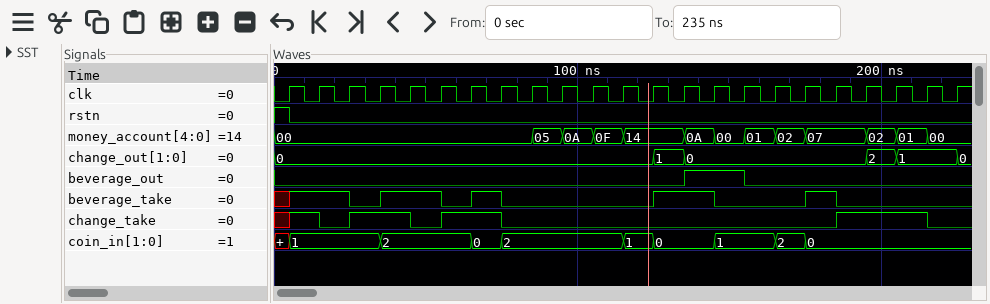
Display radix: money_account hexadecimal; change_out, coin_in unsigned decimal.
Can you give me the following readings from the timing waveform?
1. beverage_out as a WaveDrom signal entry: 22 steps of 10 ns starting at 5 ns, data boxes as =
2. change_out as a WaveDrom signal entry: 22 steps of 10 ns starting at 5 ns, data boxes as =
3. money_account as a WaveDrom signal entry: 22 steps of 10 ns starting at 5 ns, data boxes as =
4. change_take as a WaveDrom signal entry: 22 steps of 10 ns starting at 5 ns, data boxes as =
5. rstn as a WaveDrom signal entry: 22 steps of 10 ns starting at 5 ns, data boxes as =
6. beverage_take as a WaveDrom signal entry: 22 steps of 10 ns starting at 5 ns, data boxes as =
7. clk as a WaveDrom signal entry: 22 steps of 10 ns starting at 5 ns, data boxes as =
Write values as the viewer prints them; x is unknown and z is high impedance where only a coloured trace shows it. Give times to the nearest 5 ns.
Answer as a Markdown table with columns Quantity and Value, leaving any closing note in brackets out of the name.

| Quantity | Value |
|---|---|
| beverage_out as a WaveDrom signal entry: 22 steps of 10 ns starting at 5 ns, data boxes as = | {name: 'beverage_out', wave: '0............1.0......'} |
| change_out as a WaveDrom signal entry: 22 steps of 10 ns starting at 5 ns, data boxes as = | {name: 'change_out', wave: '=...........==.....==.', data: '0 1 0 2 1'} |
| money_account as a WaveDrom signal entry: 22 steps of 10 ns starting at 5 ns, data boxes as = | {name: 'money_account', wave: '=.......====.=====.===', data: '00 05 0A 0F 14 0A 00 01 02 07 02 01 00'} |
| change_take as a WaveDrom signal entry: 22 steps of 10 ns starting at 5 ns, data boxes as = | {name: 'change_take', wave: '101.01.0..........1..0'} |
| rstn as a WaveDrom signal entry: 22 steps of 10 ns starting at 5 ns, data boxes as = | {name: 'rstn', wave: '0.....................'} |
| beverage_take as a WaveDrom signal entry: 22 steps of 10 ns starting at 5 ns, data boxes as = | {name: 'beverage_take', wave: '1.01.010....1.0..10...'} |
| clk as a WaveDrom signal entry: 22 steps of 10 ns starting at 5 ns, data boxes as = | {name: 'clk', wave: 'p.....................'} |
